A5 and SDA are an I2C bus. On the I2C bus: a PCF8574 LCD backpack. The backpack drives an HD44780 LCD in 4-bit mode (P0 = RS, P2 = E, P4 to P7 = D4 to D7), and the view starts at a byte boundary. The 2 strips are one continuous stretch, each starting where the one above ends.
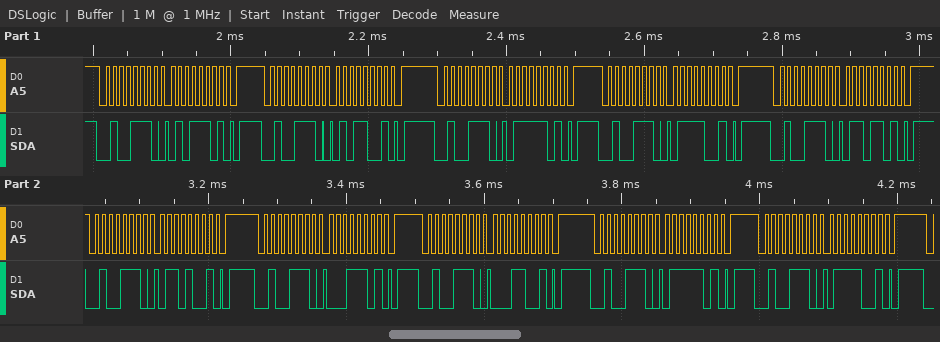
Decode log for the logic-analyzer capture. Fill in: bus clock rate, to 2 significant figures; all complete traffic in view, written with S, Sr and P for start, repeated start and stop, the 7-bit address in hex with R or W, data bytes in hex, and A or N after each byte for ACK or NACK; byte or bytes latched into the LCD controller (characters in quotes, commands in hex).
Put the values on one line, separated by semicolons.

100 kHz; S 27W A 5D A P S 27W A 59 A P S 27W A 7D A P S 27W A 79 A P S 27W A 6D A P S 27W A 69 A P S 27W A 1D A P S 27W A 19 A P S 27W A 7D A P S 27W A 79 A P; 'W' 'a'
